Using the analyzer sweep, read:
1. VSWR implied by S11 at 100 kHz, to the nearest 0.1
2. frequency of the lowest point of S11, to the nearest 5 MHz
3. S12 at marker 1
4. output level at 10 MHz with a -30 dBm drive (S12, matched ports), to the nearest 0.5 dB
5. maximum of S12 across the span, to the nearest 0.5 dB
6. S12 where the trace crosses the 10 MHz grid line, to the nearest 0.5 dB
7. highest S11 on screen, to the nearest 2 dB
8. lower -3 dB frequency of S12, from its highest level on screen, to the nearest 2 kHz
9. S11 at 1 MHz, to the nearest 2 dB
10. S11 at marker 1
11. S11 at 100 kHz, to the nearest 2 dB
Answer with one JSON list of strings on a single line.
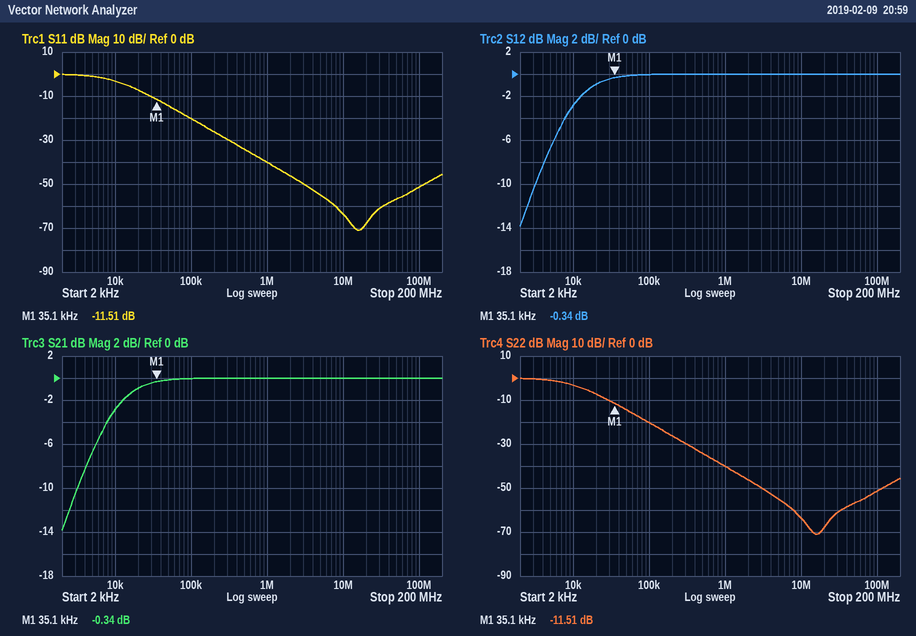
["1.2", "15 MHz", "-0.34 dB", "-30.0 dBm", "0.0 dB", "0.0 dB", "0 dB", "10 kHz", "-40 dB", "-11.51 dB", "-20 dB"]
